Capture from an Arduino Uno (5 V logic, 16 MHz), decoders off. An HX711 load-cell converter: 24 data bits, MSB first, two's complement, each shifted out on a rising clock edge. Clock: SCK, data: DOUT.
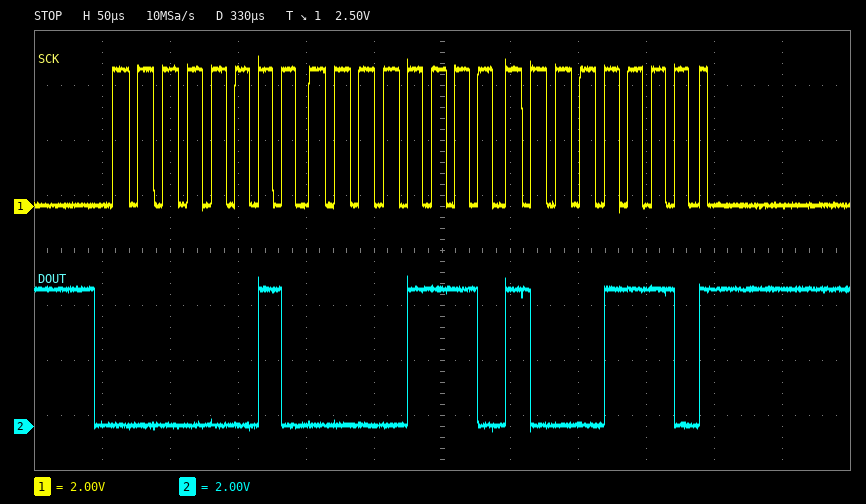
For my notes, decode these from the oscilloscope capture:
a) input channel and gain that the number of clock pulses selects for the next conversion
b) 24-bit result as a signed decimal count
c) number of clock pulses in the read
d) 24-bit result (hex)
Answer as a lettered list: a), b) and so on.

a) channel A, gain 128
b) 134798
c) 25
d) 0x020E8E
